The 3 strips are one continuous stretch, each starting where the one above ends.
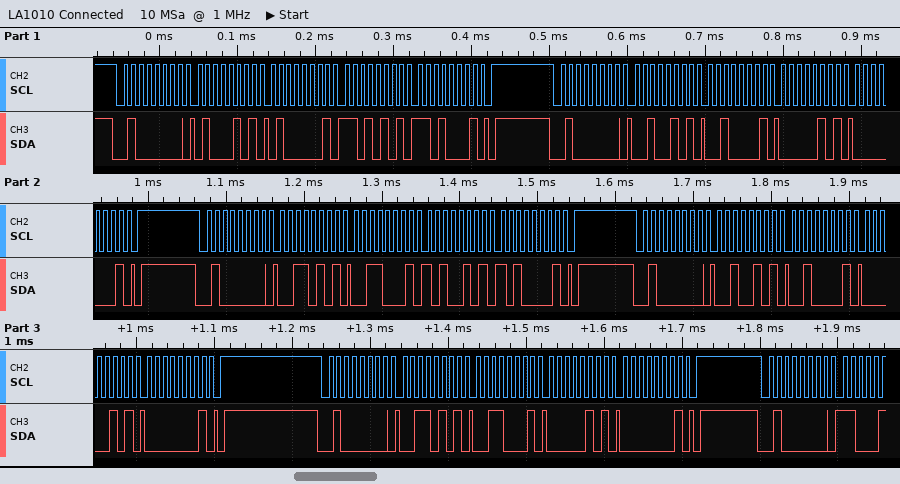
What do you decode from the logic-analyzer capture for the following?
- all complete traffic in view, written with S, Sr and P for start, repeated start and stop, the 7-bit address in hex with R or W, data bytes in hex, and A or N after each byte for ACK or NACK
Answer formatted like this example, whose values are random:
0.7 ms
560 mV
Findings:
S 20W A 45 A 41 A D5 A D1 A P S 20W A 25 A 21 A 05 A 01 A P S 20W A 35 A 31 A A5 A A1 A P S 20W A 25 A 21 A 05 A 01 A P S 20W A 35 A 31 A 05 A 01 A P S 20W A
